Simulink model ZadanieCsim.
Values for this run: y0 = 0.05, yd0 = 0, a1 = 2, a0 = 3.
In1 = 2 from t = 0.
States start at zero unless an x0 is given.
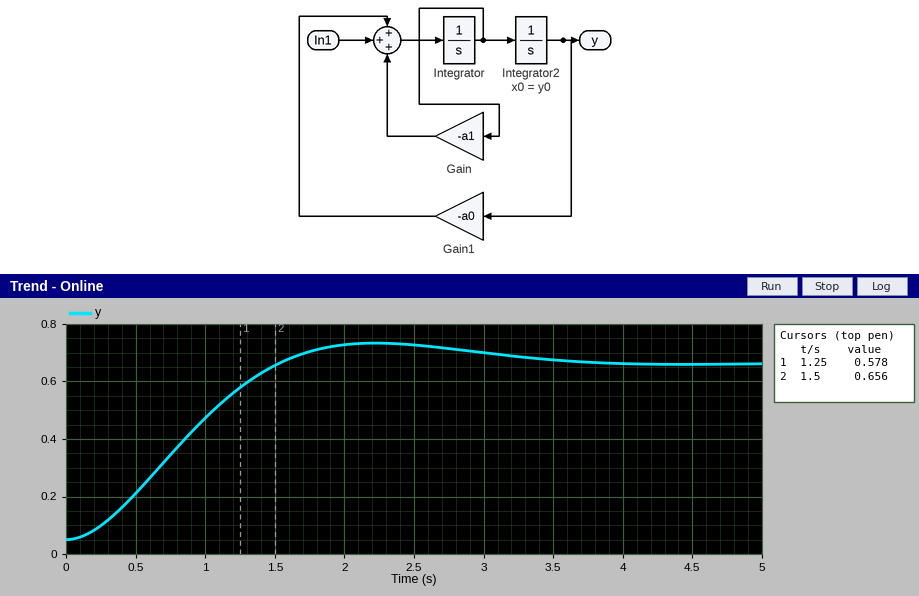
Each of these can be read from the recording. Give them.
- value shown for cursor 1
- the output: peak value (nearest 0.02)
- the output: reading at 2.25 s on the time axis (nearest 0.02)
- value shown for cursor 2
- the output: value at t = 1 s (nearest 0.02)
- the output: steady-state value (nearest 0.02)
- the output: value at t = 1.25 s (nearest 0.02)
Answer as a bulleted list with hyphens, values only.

- 0.578
- 0.74
- 0.74
- 0.656
- 0.48
- 0.66
- 0.58
